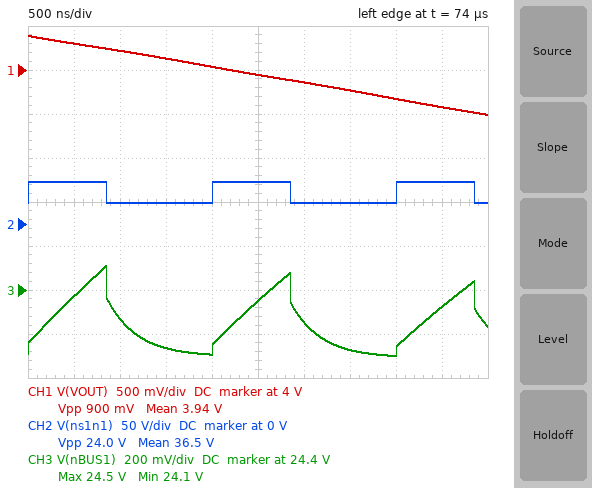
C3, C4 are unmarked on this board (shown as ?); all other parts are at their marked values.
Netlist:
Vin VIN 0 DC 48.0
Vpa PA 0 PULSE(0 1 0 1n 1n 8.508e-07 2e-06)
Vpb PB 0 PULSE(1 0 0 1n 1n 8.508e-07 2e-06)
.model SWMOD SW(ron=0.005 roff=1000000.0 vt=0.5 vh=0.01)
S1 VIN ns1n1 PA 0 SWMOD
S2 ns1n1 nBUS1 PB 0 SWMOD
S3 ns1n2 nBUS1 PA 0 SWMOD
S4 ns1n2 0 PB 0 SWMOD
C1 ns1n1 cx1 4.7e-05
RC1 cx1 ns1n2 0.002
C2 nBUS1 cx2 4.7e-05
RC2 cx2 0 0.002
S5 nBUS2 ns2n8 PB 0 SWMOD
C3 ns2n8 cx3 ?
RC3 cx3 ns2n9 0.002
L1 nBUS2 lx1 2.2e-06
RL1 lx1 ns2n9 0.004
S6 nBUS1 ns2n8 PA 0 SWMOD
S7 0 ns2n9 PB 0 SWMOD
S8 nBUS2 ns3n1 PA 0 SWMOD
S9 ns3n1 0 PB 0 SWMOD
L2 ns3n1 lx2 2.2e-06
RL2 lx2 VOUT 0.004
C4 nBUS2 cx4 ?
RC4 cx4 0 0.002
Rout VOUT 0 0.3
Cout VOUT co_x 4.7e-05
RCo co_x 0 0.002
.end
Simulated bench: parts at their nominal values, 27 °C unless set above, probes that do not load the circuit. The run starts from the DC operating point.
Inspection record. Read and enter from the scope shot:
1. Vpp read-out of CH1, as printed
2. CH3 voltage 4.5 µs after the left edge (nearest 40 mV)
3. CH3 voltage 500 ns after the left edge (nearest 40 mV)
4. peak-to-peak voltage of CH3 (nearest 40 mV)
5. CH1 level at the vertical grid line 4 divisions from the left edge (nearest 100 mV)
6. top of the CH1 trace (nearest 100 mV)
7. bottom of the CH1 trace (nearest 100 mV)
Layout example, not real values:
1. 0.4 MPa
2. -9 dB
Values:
1. 900 mV
2. 24.32 V
3. 24.36 V
4. 400 mV
5. 4.0 V
6. 4.4 V
7. 3.5 V
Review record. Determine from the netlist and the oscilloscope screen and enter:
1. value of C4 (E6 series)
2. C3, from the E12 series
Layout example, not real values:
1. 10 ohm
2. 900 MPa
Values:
1. 150 µF
2. 56 µF
